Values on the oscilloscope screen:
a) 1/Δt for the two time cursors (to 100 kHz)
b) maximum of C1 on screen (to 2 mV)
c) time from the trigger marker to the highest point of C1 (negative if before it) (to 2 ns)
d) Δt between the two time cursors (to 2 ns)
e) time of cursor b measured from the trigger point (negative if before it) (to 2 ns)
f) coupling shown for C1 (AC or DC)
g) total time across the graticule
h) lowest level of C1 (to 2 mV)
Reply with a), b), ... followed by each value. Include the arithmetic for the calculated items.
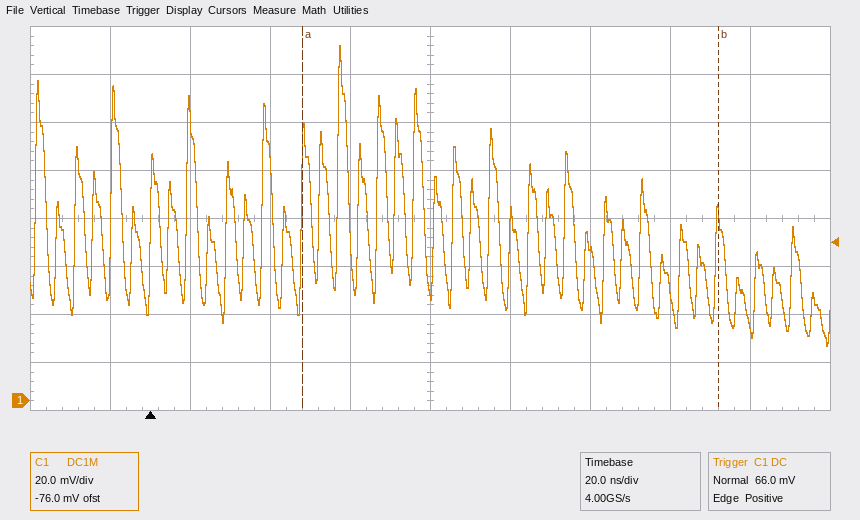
a) 1 / 104 ns ≈ 9.6 MHz
b) 148 mV
c) +48 ns
d) 104 ns
e) +142 ns
f) DC
g) 200 ns
h) 24 mV
